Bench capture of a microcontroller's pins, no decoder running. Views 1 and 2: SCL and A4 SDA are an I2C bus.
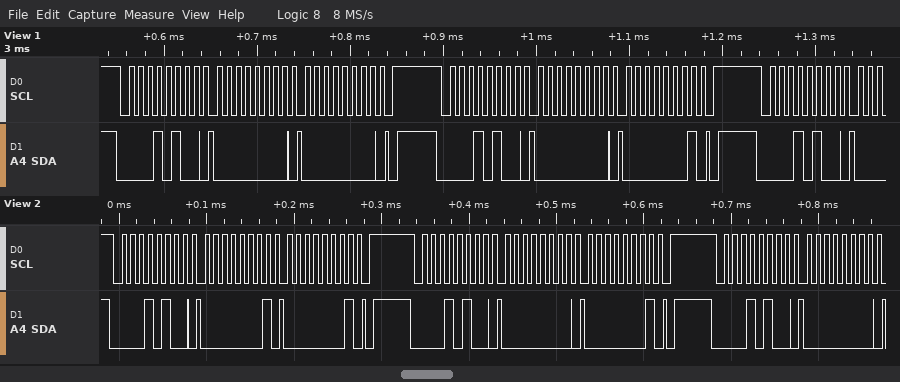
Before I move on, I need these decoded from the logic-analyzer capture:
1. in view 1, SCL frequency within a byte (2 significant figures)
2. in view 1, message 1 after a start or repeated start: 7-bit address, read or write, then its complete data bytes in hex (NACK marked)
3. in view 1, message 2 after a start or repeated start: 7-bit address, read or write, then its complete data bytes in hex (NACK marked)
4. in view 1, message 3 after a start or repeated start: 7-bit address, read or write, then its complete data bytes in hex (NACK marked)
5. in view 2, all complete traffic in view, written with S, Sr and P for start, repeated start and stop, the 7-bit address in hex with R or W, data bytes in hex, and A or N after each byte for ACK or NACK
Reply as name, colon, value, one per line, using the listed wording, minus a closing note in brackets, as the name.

in view 1, SCL frequency within a byte: 100 kHz
in view 1, message 1 after a start or repeated start: 7-bit address, read or write, then its complete data bytes in hex: 0x0A write: 00 00
in view 1, message 2 after a start or repeated start: 7-bit address, read or write, then its complete data bytes in hex: 0x0A write: 00 01
in view 1, message 3 after a start or repeated start: 7-bit address, read or write, then its complete data bytes in hex: 0x0A write
in view 2, all complete traffic in view, written with S, Sr and P for start, repeated start and stop, the 7-bit address in hex with R or W, data bytes in hex, and A or N after each byte for ACK or NACK: S 0AW A 01 A 01 A P S 0AW A 00 A 01 A P S 0AW A 00 A
